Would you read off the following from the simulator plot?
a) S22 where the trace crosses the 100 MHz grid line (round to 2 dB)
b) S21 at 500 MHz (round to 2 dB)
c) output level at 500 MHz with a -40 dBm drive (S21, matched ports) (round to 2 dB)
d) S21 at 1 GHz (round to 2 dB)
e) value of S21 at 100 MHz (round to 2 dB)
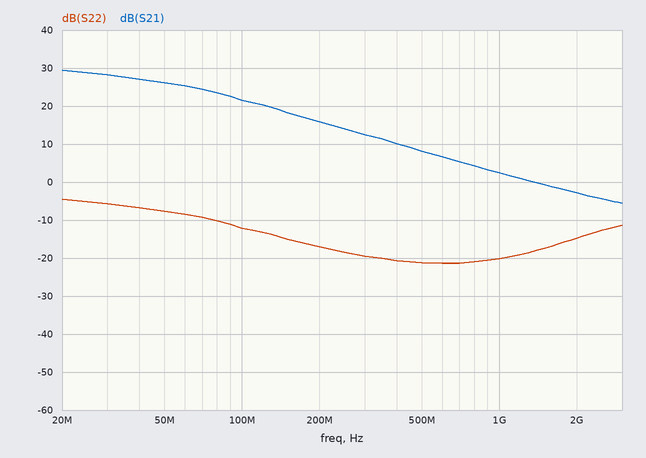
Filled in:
-12 dB
8 dB
-32 dBm
2 dB
22 dB
